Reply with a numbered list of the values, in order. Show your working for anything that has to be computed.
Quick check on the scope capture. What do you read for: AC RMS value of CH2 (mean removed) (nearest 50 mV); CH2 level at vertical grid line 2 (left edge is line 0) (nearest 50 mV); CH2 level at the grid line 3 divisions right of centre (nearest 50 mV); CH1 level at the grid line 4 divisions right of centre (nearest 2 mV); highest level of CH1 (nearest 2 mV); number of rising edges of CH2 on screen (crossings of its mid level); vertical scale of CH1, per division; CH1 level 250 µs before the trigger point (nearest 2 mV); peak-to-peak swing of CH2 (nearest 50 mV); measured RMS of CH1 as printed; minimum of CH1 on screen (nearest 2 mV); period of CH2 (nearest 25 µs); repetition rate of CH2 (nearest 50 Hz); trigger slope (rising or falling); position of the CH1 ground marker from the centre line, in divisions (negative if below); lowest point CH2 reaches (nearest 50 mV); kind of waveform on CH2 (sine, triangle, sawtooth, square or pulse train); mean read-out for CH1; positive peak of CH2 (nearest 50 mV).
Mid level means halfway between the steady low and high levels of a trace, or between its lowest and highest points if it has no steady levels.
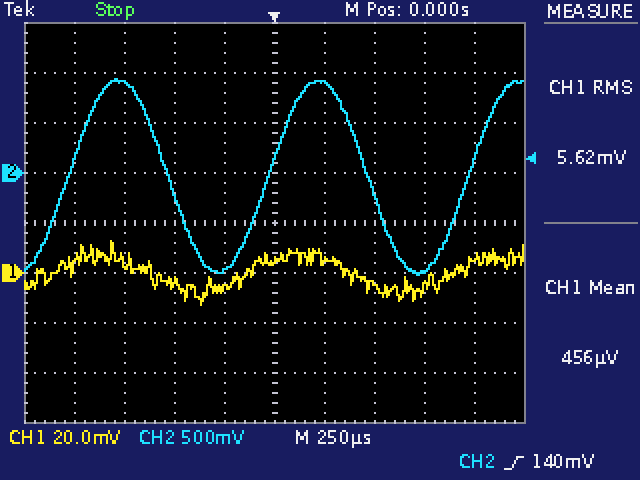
1. 1.95 V / (2√2) ≈ 689 mV, so 700 mV to the nearest 50 mV
2. 900 mV
3. -1.00 V
4. 6 mV
5. 12 mV
6. 3
7. 20 mV
8. -6 mV
9. 950 mV − (-1.00 V) = 1.95 V
10. 5.62 mV
11. -12 mV
12. 1.000 ms
13. 1 / 1.000 ms ≈ 1.00 kHz
14. rising
15. -1.0 div
16. -1.00 V
17. sine
18. 456 µV
19. 950 mV
